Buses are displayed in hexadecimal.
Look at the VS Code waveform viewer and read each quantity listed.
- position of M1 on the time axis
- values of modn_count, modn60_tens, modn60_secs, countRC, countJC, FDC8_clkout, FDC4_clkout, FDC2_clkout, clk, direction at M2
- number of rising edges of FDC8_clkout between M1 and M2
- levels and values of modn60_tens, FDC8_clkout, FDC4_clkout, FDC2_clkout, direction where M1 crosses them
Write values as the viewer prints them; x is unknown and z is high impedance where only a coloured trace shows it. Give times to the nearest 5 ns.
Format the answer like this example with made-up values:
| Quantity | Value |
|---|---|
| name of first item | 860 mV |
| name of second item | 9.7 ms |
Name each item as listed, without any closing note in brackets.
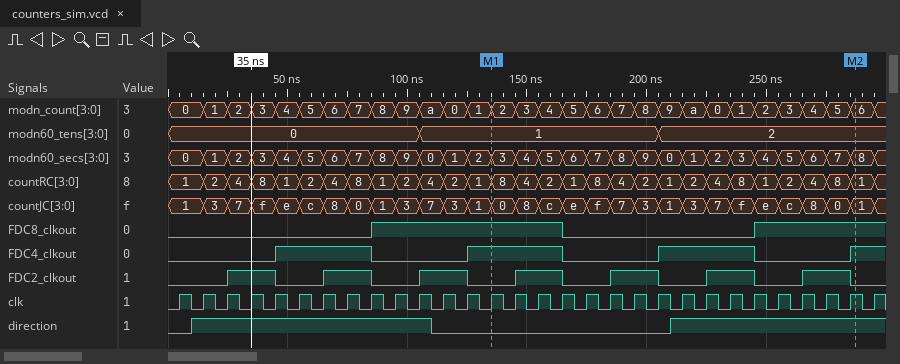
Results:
| Quantity | Value |
|---|---|
| position of M1 on the time axis | 135 ns |
| values of modn_count, modn60_tens, modn60_secs, countRC, countJC, FDC8_clkout, FDC4_clkout, FDC2_clkout, clk, direction at M2 | modn_count=6, modn60_tens=2, modn60_secs=8, countRC=1, countJC=1, FDC8_clkout=1, FDC4_clkout=1, FDC2_clkout=0, clk=1, direction=1 |
| number of rising edges of FDC8_clkout between M1 and M2 | 1 |
| levels and values of modn60_tens, FDC8_clkout, FDC4_clkout, FDC2_clkout, direction where M1 crosses them | modn60_tens=1, FDC8_clkout=1, FDC4_clkout=1, FDC2_clkout=0, direction=0 |
